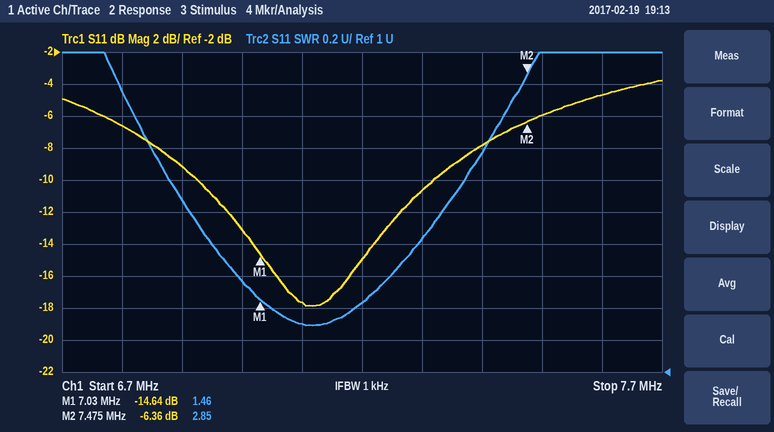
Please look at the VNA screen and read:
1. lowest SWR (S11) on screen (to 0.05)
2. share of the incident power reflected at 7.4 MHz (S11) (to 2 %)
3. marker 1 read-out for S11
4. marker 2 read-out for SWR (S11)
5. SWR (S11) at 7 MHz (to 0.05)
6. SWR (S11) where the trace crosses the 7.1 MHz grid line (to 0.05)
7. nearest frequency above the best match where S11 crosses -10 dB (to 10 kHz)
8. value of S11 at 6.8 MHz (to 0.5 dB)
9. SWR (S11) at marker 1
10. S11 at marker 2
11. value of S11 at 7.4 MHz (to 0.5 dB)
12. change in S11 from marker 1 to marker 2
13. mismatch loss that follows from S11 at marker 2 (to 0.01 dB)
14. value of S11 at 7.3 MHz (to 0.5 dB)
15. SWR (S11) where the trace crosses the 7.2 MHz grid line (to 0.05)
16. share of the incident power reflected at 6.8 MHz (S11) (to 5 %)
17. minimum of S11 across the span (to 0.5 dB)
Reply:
1.30
16 %
-14.64 dB
2.85
1.55
1.30
7.32 MHz
-6.5 dB
1.46
-6.36 dB
-8.0 dB
8.28 dB
1.14 dB
-10.5 dB
1.45
20 %
-18.0 dB
